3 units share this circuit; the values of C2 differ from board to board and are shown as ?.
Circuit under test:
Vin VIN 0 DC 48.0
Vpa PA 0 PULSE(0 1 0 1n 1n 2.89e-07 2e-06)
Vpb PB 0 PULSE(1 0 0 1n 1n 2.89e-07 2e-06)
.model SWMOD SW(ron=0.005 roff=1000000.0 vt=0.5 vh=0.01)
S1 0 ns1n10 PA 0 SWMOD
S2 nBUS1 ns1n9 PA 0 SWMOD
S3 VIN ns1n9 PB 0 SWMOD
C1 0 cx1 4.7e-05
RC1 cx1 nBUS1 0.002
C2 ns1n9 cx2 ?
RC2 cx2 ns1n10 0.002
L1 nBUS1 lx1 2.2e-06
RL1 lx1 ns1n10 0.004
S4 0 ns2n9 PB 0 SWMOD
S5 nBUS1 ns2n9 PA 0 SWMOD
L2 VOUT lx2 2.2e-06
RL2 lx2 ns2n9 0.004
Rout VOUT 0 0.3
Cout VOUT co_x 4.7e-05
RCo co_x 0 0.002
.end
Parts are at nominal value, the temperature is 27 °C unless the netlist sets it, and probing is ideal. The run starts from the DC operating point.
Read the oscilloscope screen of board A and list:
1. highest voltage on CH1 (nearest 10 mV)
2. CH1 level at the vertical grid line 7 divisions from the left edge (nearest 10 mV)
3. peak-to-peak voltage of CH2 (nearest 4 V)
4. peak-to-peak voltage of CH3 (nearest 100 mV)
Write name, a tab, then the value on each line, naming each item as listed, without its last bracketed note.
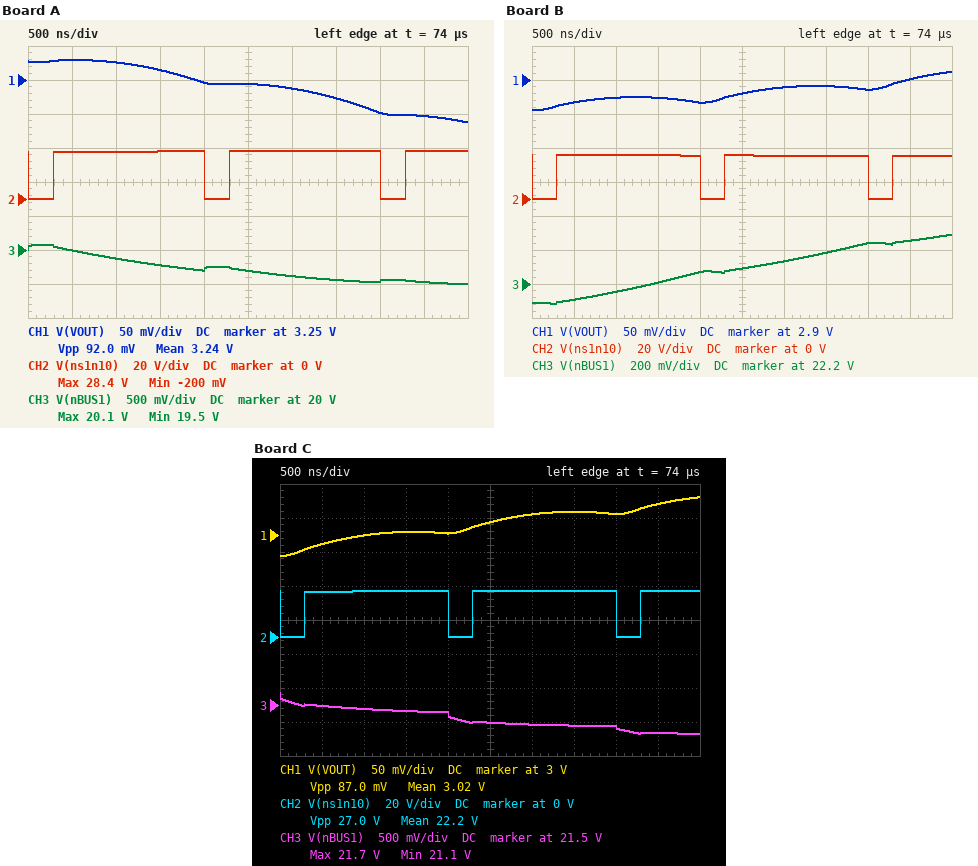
highest voltage on CH1	3.28 V
CH1 level at the vertical grid line 7 divisions from the left edge	3.22 V
peak-to-peak voltage of CH2	28 V
peak-to-peak voltage of CH3	600 mV
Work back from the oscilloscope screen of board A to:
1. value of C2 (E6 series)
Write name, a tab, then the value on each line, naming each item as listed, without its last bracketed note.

value of C2	68 µF
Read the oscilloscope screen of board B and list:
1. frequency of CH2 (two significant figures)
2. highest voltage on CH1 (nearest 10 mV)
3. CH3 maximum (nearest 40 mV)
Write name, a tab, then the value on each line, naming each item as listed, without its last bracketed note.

frequency of CH2	500 kHz
highest voltage on CH1	2.91 V
CH3 maximum	22.48 V
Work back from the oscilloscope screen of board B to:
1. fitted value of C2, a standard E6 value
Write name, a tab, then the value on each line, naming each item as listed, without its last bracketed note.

fitted value of C2, a standard E6 value	33 µF
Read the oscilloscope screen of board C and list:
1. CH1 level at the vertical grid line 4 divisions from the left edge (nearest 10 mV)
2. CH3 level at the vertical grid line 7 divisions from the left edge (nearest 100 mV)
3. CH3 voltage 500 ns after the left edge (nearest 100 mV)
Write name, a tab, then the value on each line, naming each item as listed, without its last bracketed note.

CH1 level at the vertical grid line 4 divisions from the left edge	3.00 V
CH3 level at the vertical grid line 7 divisions from the left edge	21.2 V
CH3 voltage 500 ns after the left edge	21.5 V
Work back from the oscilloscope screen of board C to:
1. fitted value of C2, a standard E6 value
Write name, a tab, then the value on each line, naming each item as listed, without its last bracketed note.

fitted value of C2, a standard E6 value	15 µF
